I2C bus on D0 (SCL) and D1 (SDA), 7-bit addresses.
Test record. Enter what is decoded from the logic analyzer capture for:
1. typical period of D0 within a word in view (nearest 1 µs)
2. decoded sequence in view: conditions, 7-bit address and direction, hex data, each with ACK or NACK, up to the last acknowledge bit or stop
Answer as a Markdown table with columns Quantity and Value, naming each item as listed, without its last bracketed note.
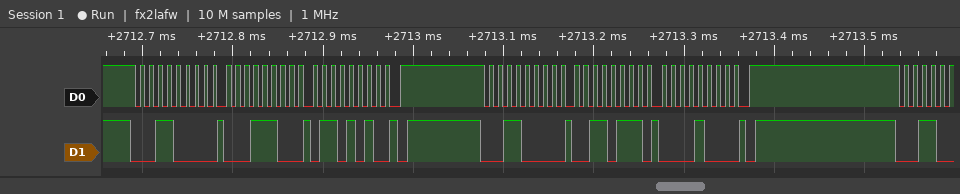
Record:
| Quantity | Value |
|---|---|
| typical period of D0 within a word in view | 10 µs |
| decoded sequence in view: conditions, 7-bit address and direction, hex data, each with ACK or NACK, up to the last acknowledge bit or stop | start, address 18 write ACK, 1C ACK, 6A ACK, stop, start, address 18 write ACK, 37 ACK, 08 ACK, stop |
